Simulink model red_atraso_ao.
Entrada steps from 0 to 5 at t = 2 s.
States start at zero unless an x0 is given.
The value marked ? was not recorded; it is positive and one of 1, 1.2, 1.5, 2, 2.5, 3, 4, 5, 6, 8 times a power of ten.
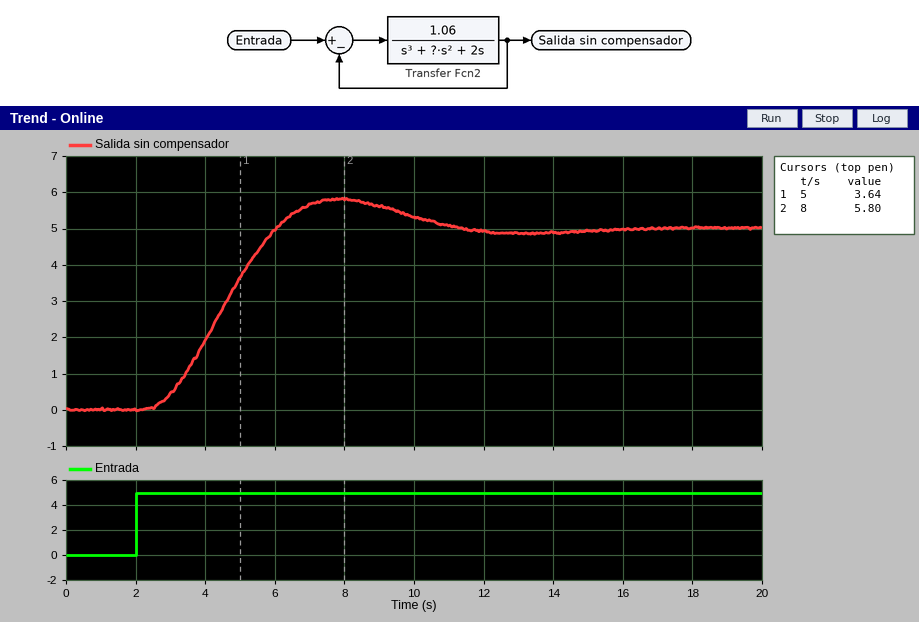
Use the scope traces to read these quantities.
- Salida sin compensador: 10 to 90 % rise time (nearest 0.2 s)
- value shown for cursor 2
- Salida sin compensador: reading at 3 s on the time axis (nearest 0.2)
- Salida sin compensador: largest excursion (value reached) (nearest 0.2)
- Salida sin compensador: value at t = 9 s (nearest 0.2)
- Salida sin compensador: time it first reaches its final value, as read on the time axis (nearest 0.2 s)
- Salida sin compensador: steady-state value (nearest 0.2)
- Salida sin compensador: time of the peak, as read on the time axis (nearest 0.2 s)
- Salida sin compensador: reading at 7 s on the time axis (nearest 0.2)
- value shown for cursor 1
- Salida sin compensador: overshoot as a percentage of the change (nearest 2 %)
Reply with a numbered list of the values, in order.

1. 2.6 s
2. 5.80
3. 0.4
4. 5.8
5. 5.6
6. 6.0 s
7. 5.0
8. 7.8 s
9. 5.6
10. 3.64
11. 16 %
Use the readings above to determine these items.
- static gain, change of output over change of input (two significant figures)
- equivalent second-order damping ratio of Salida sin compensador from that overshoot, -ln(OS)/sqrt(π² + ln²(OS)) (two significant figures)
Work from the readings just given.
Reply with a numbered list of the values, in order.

1. 1.0
2. 0.50
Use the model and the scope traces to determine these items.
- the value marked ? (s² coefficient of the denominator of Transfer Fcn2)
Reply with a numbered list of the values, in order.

1. 3
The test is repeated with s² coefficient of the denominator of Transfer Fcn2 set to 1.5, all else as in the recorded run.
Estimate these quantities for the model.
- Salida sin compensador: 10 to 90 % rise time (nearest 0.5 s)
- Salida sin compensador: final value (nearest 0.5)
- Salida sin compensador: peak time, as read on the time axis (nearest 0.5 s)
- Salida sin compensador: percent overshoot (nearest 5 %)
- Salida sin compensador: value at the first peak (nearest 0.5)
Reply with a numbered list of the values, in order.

1. 2.0 s
2. 5.0
3. 6.0 s
4. 10 %
5. 5.5
